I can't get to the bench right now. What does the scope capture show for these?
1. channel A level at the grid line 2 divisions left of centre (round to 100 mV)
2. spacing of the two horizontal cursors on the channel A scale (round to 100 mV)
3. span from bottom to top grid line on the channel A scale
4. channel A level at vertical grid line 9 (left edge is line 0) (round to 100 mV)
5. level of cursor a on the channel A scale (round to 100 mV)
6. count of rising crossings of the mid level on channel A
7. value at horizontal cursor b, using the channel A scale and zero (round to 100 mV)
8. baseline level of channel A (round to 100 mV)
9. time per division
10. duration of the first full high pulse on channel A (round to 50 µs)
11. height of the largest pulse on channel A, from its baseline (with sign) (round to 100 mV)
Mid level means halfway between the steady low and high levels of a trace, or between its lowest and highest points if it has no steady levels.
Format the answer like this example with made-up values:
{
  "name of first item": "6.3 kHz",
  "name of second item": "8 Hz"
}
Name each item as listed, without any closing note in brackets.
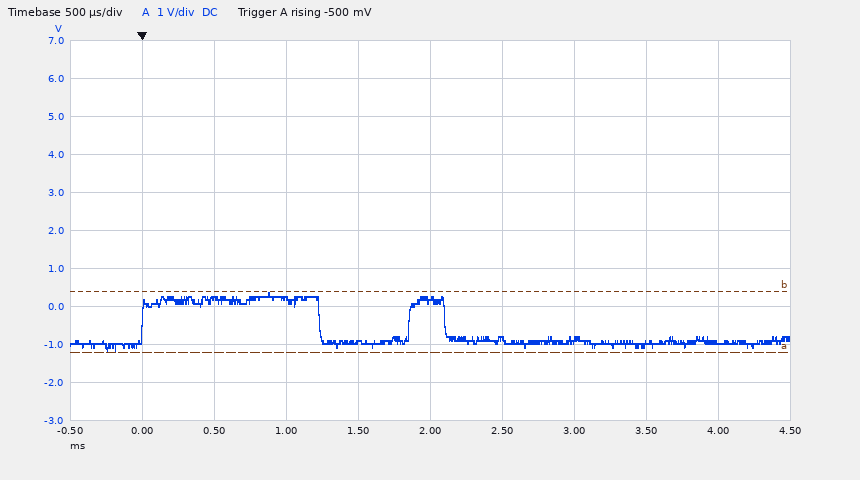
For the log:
{
  "channel A level at the grid line 2 divisions left of centre": "200 mV",
  "spacing of the two horizontal cursors on the channel A scale": "1.6 V",
  "span from bottom to top grid line on the channel A scale": "10 V",
  "channel A level at vertical grid line 9 (left edge is line 0)": "-900 mV",
  "level of cursor a on the channel A scale": "-1.2 V",
  "count of rising crossings of the mid level on channel A": "2",
  "value at horizontal cursor b, using the channel A scale and zero": "400 mV",
  "baseline level of channel A": "-900 mV",
  "time per division": "500 µs",
  "duration of the first full high pulse on channel A": "1.25 ms",
  "height of the largest pulse on channel A, from its baseline (with sign)": "+1.3 V"
}
